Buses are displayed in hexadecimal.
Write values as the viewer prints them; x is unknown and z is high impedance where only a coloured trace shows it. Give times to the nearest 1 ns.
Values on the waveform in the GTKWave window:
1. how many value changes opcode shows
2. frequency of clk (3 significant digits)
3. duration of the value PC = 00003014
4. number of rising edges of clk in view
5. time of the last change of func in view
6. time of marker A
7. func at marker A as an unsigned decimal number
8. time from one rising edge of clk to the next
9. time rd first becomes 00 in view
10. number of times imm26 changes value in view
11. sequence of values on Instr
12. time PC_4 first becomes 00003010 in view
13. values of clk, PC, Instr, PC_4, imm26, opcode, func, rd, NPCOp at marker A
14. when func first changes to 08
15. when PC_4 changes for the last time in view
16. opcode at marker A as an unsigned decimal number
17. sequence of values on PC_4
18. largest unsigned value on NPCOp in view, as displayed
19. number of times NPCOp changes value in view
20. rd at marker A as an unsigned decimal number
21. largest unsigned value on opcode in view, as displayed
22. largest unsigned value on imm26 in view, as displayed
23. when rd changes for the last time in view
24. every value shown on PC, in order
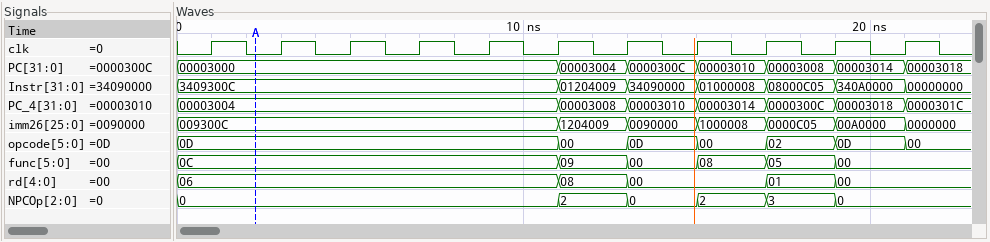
6
500 MHz
2 ns
11
19 ns
2 ns
12
2 ns
13 ns
6
3409300C, 01204009, 34090000, 01000008, 08000C05, 340A0000, 00000000
13 ns
clk=0, PC=00003000, Instr=3409300C, PC_4=00003004, imm26=009300C, opcode=0D, func=0C, rd=06, NPCOp=0
15 ns
21 ns
13
00003004, 00003008, 00003010, 00003014, 0000300C, 00003018, 0000301C
3
5
6
0D
1204009
19 ns
00003000, 00003004, 0000300C, 00003010, 00003008, 00003014, 00003018
